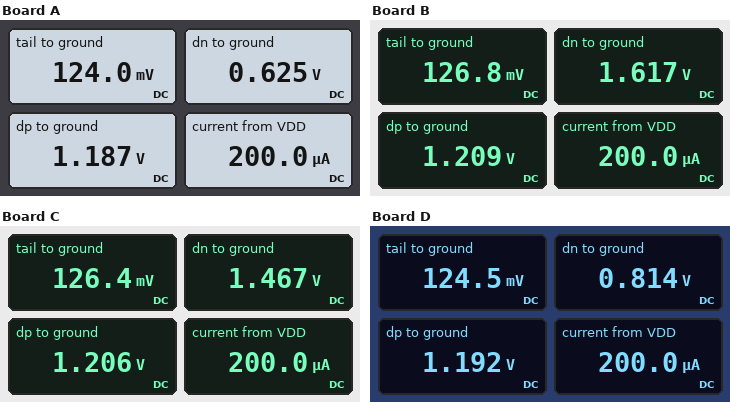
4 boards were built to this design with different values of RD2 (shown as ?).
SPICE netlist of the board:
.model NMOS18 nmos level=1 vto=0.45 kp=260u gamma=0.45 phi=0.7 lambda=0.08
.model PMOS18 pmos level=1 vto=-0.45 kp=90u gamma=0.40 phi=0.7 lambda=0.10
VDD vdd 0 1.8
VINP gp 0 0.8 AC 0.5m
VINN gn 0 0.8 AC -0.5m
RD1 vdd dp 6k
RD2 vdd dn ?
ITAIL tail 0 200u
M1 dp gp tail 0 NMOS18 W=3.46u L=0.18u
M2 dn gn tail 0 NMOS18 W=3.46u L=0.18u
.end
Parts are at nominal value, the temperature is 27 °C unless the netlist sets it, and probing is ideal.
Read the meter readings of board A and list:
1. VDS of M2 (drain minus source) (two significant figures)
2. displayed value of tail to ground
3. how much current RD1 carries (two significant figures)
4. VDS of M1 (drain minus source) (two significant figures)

500 mV
124.0 mV
100 µA
1.1 V
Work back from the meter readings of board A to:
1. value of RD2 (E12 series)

12 kΩ
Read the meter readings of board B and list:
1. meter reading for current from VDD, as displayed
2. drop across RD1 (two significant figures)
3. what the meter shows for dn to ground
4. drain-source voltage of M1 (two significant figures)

200.0 µA
590 mV
1.617 V
1.1 V
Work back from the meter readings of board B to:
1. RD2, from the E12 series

1.8 kΩ
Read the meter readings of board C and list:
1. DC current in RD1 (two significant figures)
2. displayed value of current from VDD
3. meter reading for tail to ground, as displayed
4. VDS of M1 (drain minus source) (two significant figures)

99 µA
200.0 µA
126.4 mV
1.1 V
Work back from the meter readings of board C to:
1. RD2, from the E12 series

3.3 kΩ
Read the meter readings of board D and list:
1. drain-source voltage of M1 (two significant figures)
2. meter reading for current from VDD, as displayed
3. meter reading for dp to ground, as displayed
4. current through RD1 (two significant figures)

1.1 V
200.0 µA
1.192 V
100 µA
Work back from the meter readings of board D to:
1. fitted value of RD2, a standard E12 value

10 kΩ
